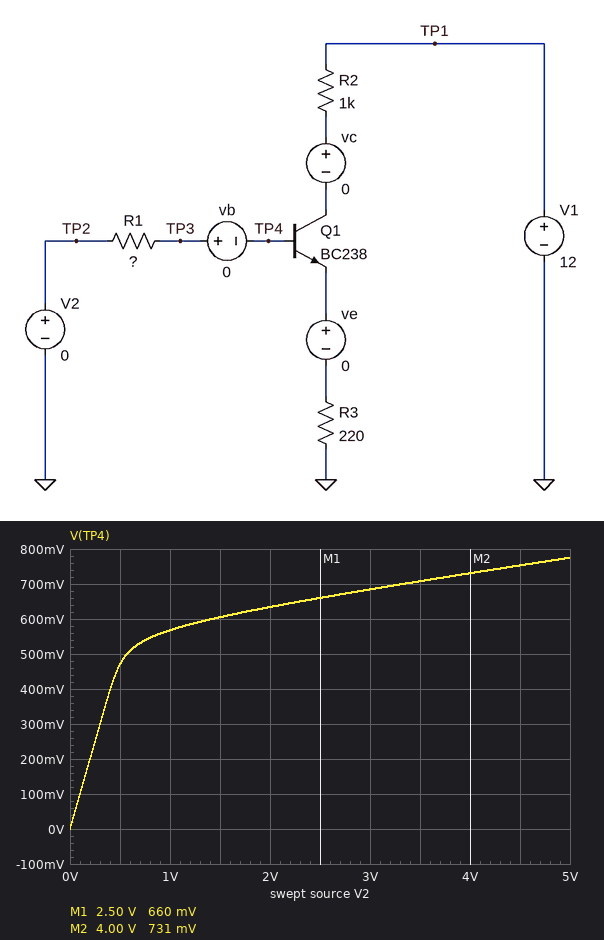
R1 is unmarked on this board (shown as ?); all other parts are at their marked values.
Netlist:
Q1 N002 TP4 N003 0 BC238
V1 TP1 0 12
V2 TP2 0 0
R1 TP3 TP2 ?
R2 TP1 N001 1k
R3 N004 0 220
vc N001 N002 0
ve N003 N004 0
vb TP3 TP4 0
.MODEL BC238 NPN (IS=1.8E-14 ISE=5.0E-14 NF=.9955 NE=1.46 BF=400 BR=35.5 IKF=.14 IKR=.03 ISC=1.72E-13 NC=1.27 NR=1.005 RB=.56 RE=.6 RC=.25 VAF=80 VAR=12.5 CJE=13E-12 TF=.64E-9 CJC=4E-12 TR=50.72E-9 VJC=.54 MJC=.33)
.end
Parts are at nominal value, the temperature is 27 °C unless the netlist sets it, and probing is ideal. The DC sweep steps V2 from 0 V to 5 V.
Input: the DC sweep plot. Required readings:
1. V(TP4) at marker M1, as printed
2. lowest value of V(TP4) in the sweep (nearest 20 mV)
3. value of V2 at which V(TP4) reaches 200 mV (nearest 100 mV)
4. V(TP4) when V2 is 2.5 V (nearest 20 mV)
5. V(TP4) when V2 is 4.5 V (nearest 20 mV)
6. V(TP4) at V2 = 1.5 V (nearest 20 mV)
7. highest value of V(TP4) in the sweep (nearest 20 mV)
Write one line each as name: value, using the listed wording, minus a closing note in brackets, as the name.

V(TP4) at marker M1, as printed: 660 mV
lowest value of V(TP4) in the sweep: 0 V
value of V2 at which V(TP4) reaches 200 mV: 200 mV
V(TP4) when V2 is 2.5 V: 660 mV
V(TP4) when V2 is 4.5 V: 760 mV
V(TP4) at V2 = 1.5 V: 600 mV
highest value of V(TP4) in the sweep: 780 mV
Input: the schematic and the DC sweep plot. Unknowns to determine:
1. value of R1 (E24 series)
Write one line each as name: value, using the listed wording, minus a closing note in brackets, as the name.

value of R1: 1.8 MΩ
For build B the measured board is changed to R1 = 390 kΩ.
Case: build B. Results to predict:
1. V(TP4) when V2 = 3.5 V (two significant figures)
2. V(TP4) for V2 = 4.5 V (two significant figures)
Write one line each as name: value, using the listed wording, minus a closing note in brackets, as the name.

V(TP4) when V2 = 3.5 V: 1.1 V
V(TP4) for V2 = 4.5 V: 1.2 V
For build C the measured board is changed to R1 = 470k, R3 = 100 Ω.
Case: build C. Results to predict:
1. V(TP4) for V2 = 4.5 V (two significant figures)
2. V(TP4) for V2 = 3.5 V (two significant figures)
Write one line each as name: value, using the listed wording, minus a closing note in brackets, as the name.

V(TP4) for V2 = 4.5 V: 900 mV
V(TP4) for V2 = 3.5 V: 830 mV
